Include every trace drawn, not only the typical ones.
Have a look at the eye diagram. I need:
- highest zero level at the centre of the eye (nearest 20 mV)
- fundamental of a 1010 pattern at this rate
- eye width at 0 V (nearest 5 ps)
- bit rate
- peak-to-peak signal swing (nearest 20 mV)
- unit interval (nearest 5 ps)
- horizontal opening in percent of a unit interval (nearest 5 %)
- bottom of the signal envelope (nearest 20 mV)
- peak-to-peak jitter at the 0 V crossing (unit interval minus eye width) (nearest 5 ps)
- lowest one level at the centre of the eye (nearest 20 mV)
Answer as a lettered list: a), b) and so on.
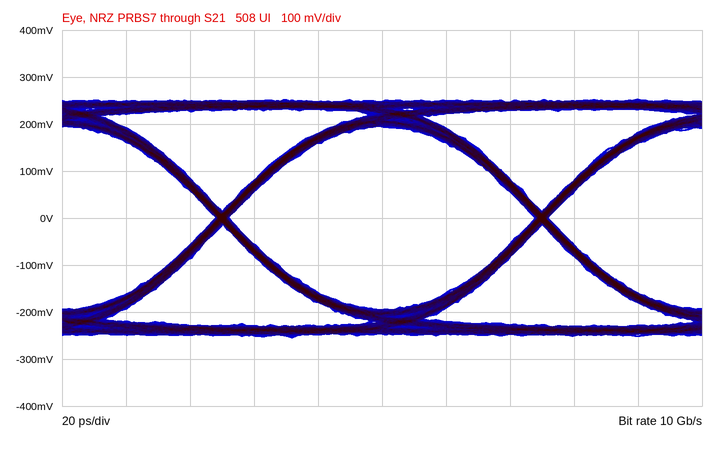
a) -200 mV
b) 5 GHz
c) 95 ps
d) 10 Gb/s
e) 500 mV
f) 100 ps
g) 95 %
h) -260 mV
i) 5 ps
j) 200 mV
